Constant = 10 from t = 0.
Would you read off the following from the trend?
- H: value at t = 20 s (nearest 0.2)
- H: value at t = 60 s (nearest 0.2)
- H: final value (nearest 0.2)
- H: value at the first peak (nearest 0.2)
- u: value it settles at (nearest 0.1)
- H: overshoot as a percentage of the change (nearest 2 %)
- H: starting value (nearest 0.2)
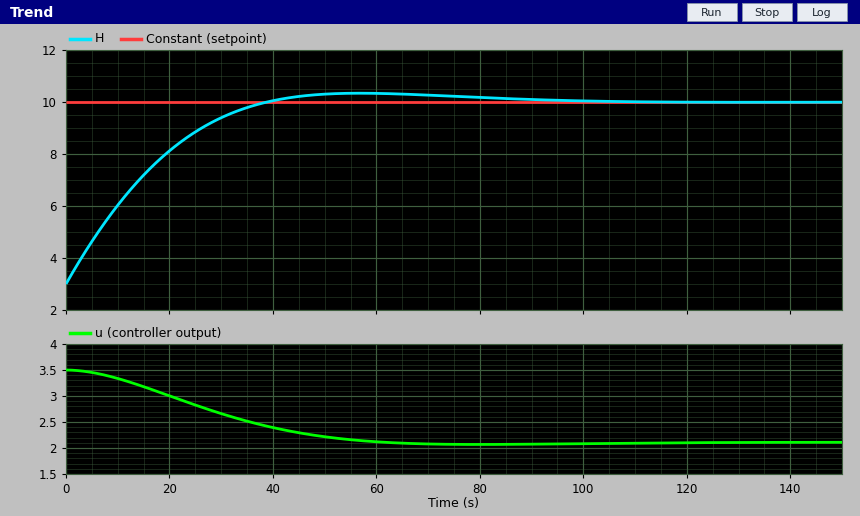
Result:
8.2
10.4
10.0
10.4
2.1
4 %
3.0
